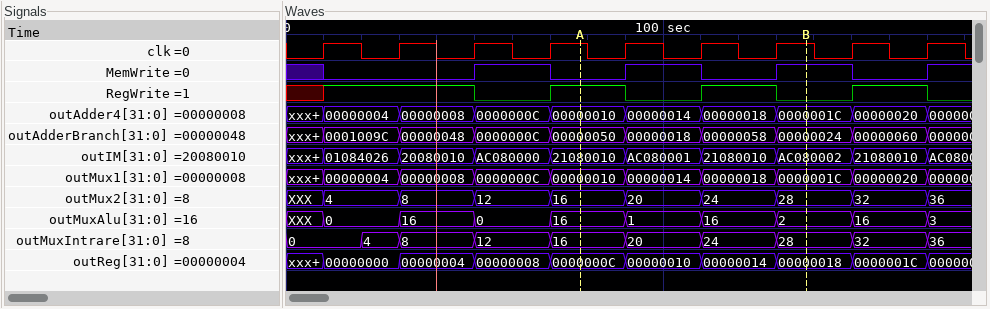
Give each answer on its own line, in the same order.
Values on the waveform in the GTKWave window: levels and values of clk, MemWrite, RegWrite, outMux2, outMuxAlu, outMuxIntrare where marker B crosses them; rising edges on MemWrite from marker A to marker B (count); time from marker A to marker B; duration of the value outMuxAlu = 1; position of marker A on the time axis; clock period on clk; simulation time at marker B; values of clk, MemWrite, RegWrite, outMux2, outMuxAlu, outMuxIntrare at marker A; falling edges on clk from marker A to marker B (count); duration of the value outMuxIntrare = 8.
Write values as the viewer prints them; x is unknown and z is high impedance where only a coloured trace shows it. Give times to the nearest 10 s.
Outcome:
clk=1, MemWrite=1, RegWrite=0, outMux2=28, outMuxAlu=2, outMuxIntrare=28
2
60 s
20 s
80 s
20 s
140 s
clk=1, MemWrite=0, RegWrite=1, outMux2=16, outMuxAlu=16, outMuxIntrare=16
3
20 s
